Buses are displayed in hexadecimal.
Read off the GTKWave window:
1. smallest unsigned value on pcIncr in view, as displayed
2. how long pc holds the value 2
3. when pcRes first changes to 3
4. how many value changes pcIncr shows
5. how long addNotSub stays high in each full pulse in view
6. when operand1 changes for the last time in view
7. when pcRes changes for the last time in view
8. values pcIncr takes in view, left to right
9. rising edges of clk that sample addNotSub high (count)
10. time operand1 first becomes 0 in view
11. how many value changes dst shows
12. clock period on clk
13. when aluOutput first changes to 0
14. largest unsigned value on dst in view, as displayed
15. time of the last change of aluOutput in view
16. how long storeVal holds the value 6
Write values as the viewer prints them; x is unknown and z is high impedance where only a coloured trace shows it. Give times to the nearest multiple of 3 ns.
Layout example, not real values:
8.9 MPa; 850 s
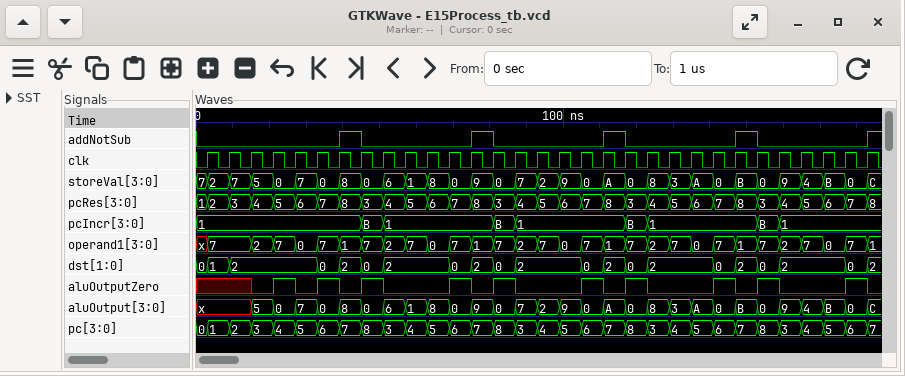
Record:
1; 6 ns; 9 ns; 8; 6 ns, 6 ns, 6 ns, 6 ns; 183 ns; 183 ns; 1, B, 1, B, 1, B, 1, B, 1; 4; 27 ns; 20; 6 ns; 21 ns; 2; 183 ns; 6 ns
